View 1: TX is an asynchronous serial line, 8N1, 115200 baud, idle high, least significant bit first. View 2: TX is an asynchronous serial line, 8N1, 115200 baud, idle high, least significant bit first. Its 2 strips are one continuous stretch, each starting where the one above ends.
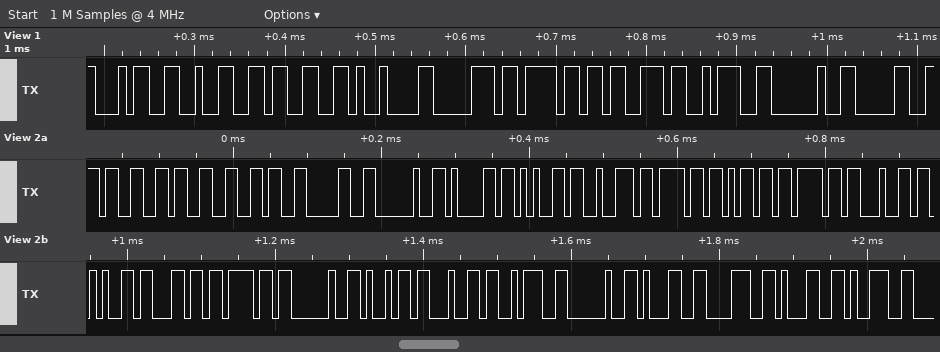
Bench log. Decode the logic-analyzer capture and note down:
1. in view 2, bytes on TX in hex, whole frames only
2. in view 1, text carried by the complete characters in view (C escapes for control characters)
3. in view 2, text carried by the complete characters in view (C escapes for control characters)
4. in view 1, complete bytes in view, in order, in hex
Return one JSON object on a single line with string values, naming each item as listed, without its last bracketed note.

{"in view 2, bytes on TX in hex, whole frames only": "33 33 36 30 20 61 65 72 6F 6D 6F 64 65 6C 6F 20 69 64 3A 20 31 38 31 39", "in view 1, text carried by the complete characters in view": "\"423\\tpos: 0\"", "in view 2, text carried by the complete characters in view": "\"3360 aeromodelo id: 1819\"", "in view 1, complete bytes in view, in order, in hex": "34 32 33 09 70 6F 73 3A 20 30"}
